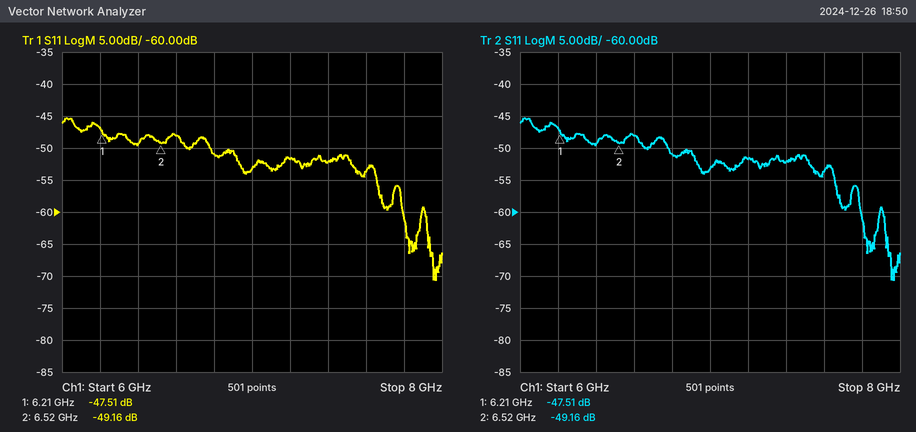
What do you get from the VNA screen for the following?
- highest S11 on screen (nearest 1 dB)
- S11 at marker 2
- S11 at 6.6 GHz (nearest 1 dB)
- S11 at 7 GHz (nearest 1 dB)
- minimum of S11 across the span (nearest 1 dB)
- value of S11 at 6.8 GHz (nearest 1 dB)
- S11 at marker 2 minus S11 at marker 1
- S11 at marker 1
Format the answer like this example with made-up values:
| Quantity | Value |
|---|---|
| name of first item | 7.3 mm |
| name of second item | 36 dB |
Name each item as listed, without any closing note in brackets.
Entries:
| Quantity | Value |
|---|---|
| highest S11 on screen | -45 dB |
| S11 at marker 2 | -49.16 dB |
| S11 at 6.6 GHz | -48 dB |
| S11 at 7 GHz | -53 dB |
| minimum of S11 across the span | -71 dB |
| value of S11 at 6.8 GHz | -51 dB |
| S11 at marker 2 minus S11 at marker 1 | -1.65 dB |
| S11 at marker 1 | -47.51 dB |
